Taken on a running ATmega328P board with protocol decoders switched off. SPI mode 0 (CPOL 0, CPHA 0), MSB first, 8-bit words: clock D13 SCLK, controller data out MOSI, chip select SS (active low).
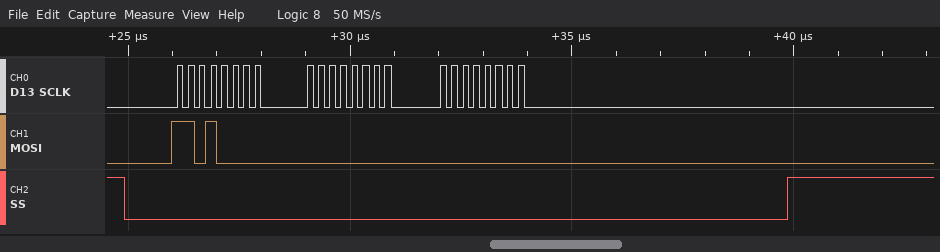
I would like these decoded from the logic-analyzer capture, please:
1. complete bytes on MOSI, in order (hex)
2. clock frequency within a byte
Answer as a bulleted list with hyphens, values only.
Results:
- 0xD0 0x00 0x00
- 4 MHz
